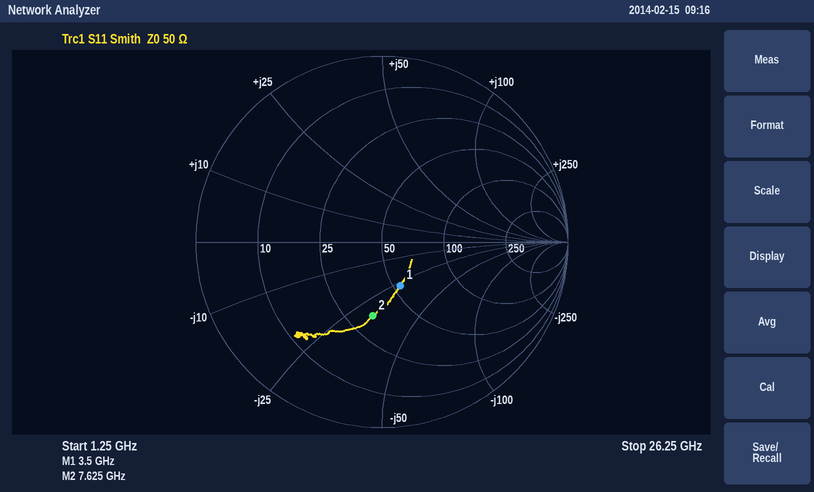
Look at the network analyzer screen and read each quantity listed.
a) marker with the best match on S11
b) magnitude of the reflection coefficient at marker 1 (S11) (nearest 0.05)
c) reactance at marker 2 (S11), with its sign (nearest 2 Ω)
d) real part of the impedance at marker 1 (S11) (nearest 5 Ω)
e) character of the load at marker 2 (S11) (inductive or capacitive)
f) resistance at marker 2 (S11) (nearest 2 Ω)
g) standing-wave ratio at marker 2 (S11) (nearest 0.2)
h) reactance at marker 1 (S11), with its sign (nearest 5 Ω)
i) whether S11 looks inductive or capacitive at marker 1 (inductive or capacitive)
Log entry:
marker 1
0.25
-32 Ω
55 Ω
capacitive
34 Ω
2.4
-25 Ω
capacitive
